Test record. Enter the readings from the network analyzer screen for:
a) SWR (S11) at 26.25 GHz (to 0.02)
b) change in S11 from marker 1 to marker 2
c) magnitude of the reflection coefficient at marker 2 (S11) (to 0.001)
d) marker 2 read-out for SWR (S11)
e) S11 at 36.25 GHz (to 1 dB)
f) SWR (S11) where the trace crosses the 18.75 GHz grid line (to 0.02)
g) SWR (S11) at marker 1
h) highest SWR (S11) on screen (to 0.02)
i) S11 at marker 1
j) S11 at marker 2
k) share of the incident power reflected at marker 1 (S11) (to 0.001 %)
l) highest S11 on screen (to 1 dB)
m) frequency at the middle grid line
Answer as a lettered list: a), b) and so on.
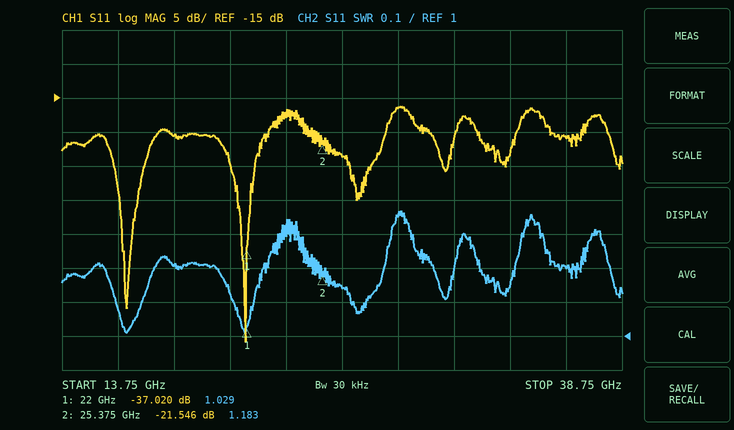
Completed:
a) 1.14
b) 15.474 dB
c) 0.084
d) 1.183
e) -21 dB
f) 1.20
g) 1.029
h) 1.36
i) -37.020 dB
j) -21.546 dB
k) 0.020 %
l) -16 dB
m) 26.25 GHz
